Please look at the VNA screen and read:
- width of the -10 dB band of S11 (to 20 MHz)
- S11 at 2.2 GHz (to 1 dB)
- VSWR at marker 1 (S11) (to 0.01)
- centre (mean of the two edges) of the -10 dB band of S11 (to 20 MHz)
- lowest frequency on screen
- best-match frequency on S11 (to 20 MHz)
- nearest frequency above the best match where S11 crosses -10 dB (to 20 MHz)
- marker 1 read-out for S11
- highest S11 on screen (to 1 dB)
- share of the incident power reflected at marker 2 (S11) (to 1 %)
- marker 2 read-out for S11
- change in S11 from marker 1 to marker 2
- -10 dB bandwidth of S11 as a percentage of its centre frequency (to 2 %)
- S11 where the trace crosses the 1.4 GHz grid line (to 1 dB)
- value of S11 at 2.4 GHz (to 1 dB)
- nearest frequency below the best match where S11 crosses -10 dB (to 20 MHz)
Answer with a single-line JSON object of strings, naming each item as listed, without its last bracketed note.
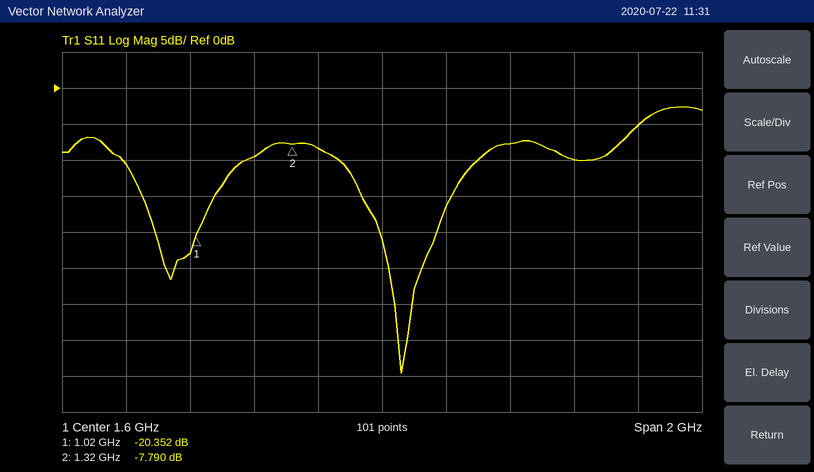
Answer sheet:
{"width of the -10 dB band of S11": "440 MHz", "S11 at 2.2 GHz": "-10 dB", "VSWR at marker 1 (S11)": "1.21", "centre (mean of the two edges) of the -10 dB band of S11": "1.68 GHz", "lowest frequency on screen": "600 MHz", "best-match frequency on S11": "1.66 GHz", "nearest frequency above the best match where S11 crosses -10 dB": "1.90 GHz", "marker 1 read-out for S11": "-20.352 dB", "highest S11 on screen": "-3 dB", "share of the incident power reflected at marker 2 (S11)": "17 %", "marker 2 read-out for S11": "-7.790 dB", "change in S11 from marker 1 to marker 2": "12.562 dB", "-10 dB bandwidth of S11 as a percentage of its centre frequency": "26 %", "S11 where the trace crosses the 1.4 GHz grid line": "-8 dB", "value of S11 at 2.4 GHz": "-5 dB", "nearest frequency below the best match where S11 crosses -10 dB": "1.46 GHz"}
